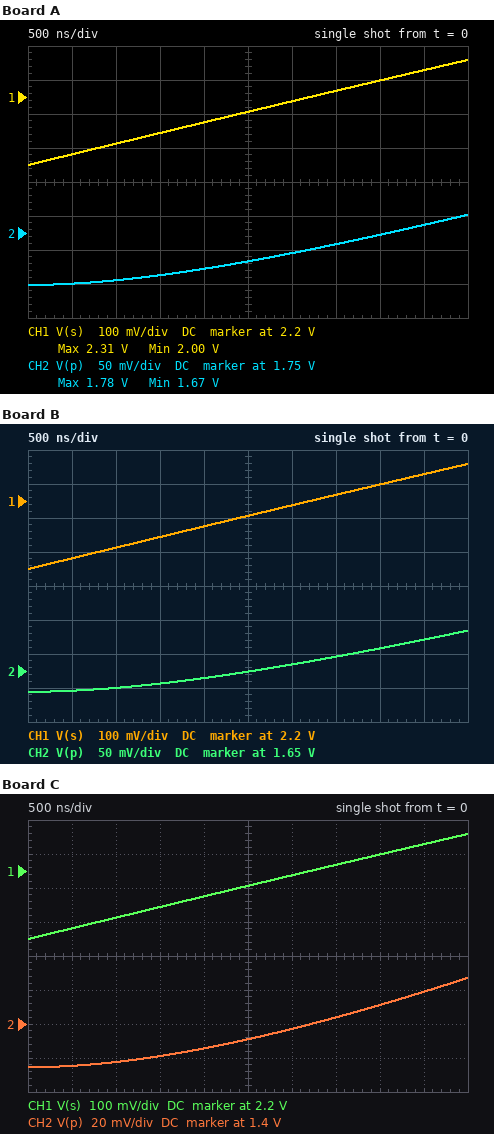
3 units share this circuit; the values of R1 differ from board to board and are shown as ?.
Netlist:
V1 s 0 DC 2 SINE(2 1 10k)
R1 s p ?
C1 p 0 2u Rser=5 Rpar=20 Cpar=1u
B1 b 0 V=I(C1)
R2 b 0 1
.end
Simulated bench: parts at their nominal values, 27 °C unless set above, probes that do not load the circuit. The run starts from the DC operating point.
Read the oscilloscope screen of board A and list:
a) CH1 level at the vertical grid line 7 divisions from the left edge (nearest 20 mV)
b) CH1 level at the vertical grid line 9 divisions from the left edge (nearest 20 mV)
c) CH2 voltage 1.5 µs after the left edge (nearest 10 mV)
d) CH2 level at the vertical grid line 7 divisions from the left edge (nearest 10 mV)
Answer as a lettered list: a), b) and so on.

a) 2.22 V
b) 2.28 V
c) 1.69 V
d) 1.73 V
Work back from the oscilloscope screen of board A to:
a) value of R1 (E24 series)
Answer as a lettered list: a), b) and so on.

a) 3.9 Ω
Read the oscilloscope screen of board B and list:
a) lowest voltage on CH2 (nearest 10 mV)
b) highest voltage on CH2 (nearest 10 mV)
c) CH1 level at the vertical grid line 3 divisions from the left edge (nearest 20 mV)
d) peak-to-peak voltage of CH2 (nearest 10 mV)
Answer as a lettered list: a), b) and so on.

a) 1.62 V
b) 1.71 V
c) 2.10 V
d) 90 mV
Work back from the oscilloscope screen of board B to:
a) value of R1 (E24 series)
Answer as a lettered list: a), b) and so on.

a) 4.7 Ω
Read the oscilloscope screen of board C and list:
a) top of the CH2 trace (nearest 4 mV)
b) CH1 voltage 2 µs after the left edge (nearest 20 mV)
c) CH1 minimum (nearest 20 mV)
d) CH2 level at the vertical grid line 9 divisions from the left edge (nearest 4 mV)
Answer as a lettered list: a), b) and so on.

a) 1.428 V
b) 2.12 V
c) 2.00 V
d) 1.420 V
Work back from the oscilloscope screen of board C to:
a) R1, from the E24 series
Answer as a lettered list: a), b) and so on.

a) 9.1 Ω
